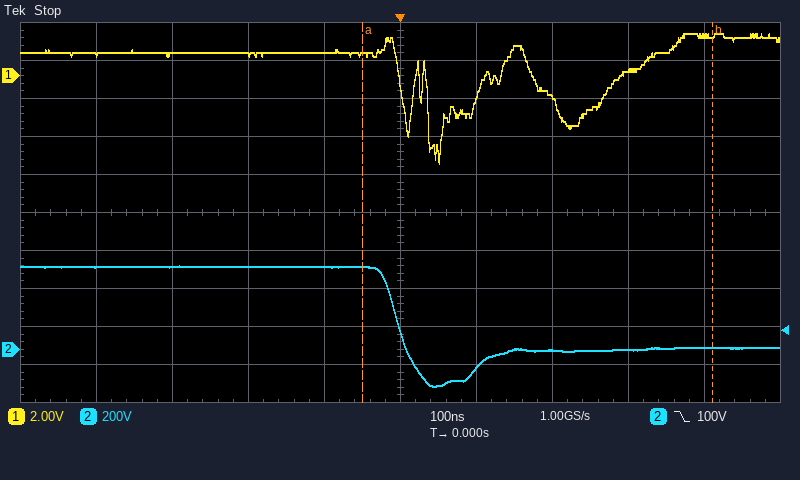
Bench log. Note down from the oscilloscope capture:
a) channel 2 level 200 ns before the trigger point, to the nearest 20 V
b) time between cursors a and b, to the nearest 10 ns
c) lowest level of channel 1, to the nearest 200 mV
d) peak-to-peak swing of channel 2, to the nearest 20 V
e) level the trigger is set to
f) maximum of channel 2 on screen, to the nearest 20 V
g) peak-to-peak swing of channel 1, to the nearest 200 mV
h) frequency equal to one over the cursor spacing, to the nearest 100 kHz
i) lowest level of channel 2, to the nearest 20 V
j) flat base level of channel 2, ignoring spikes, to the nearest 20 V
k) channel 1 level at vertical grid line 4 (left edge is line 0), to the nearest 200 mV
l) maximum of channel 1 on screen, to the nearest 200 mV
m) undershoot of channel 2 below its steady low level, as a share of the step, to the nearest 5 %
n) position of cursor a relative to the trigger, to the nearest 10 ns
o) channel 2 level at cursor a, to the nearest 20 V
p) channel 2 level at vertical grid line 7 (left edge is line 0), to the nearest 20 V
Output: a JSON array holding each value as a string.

["440 V", "460 ns", "-4.6 V", "640 V", "100 V", "440 V", "6.8 V", "2.2 MHz", "-200 V", "0 V", "1.2 V", "2.2 V", "45 %", "-50 ns", "440 V", "0 V"]
